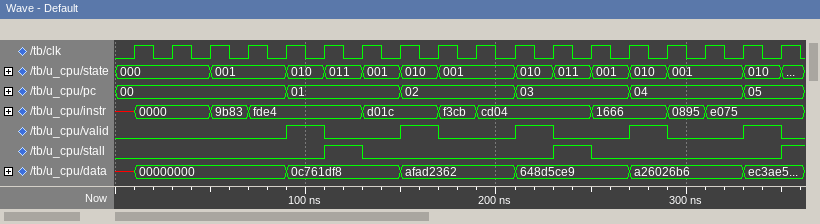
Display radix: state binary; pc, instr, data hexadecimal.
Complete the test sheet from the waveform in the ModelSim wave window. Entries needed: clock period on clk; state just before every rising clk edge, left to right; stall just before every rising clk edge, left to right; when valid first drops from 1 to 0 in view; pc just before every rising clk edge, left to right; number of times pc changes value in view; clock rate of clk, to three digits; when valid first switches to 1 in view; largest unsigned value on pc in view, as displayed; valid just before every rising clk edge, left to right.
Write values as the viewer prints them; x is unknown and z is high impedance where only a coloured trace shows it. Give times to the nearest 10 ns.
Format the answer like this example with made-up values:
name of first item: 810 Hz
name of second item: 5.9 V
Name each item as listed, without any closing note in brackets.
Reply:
clock period on clk: 20 ns
state just before every rising clk edge, left to right: 000, 000, 000, 001, 001, 010, 011, 001, 010, 001, 001, 010, 011, 001, 010, 001, 001, 010
stall just before every rising clk edge, left to right: 0 0 0 0 0 0 1 0 0 0 0 0 1 0 0 0 0 0
when valid first drops from 1 to 0 in view: 110 ns
pc just before every rising clk edge, left to right: 00, 00, 00, 00, 00, 01, 01, 01, 02, 02, 02, 03, 03, 03, 04, 04, 04, 05
number of times pc changes value in view: 5
clock rate of clk, to three digits: 50.0 MHz
when valid first switches to 1 in view: 90 ns
largest unsigned value on pc in view, as displayed: 05
valid just before every rising clk edge, left to right: 0 0 0 0 0 1 0 0 1 0 0 1 0 0 1 0 0 1
